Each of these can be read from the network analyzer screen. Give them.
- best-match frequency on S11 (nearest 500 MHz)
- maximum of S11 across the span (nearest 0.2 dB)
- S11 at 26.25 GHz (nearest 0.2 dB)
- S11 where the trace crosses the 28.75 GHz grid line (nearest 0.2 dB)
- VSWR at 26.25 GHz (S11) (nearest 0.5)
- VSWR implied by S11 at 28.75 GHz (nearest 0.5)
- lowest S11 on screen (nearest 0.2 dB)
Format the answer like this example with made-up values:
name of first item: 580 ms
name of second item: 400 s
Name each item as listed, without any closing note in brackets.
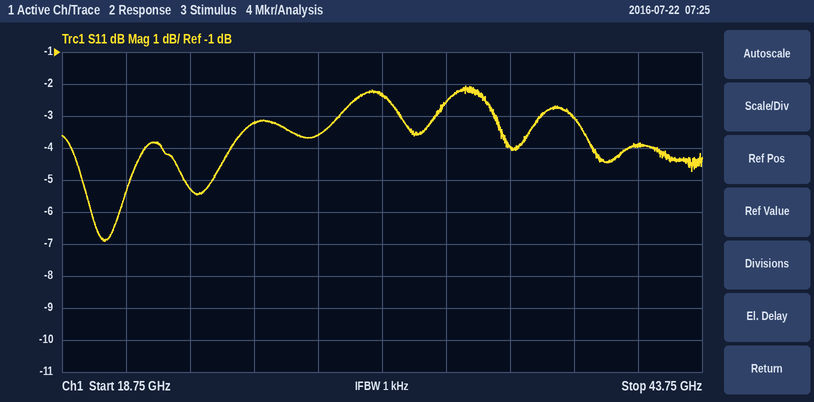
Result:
best-match frequency on S11: 20.5 GHz
maximum of S11 across the span: -2.0 dB
S11 at 26.25 GHz: -3.2 dB
S11 where the trace crosses the 28.75 GHz grid line: -3.6 dB
VSWR at 26.25 GHz (S11): 5.5
VSWR implied by S11 at 28.75 GHz: 5.0
lowest S11 on screen: -7.0 dB
